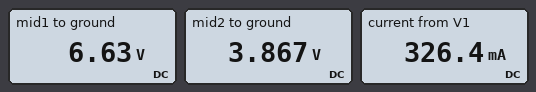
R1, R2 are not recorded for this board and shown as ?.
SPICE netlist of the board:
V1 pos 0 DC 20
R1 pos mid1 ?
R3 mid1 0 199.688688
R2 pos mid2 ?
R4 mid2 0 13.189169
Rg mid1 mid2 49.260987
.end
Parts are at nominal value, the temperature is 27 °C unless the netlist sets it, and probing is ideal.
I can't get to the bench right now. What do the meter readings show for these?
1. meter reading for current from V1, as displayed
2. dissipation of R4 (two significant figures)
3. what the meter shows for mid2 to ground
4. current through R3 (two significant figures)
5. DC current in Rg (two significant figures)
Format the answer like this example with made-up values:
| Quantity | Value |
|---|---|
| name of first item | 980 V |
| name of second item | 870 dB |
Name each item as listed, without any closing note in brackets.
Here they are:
| Quantity | Value |
|---|---|
| meter reading for current from V1, as displayed | 326.4 mA |
| dissipation of R4 | 1.1 W |
| what the meter shows for mid2 to ground | 3.867 V |
| current through R3 | 33 mA |
| DC current in Rg | 56 mA |
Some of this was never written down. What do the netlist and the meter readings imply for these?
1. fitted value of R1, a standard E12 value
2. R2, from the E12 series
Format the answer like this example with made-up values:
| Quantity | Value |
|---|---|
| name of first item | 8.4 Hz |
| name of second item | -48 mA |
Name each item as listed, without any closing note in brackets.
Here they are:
| Quantity | Value |
|---|---|
| fitted value of R1, a standard E12 value | 150 Ω |
| R2, from the E12 series | 68 Ω |
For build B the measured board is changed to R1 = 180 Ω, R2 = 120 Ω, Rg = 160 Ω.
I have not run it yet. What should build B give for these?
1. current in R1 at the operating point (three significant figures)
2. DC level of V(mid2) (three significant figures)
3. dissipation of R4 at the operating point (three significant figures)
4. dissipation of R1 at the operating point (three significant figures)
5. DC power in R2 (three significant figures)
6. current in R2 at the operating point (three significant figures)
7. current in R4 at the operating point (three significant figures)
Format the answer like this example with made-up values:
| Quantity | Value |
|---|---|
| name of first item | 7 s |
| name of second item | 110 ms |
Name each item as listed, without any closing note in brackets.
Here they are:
| Quantity | Value |
|---|---|
| current in R1 at the operating point | 69.5 mA |
| DC level of V(mid2) | 2.36 V |
| dissipation of R4 at the operating point | 423 mW |
| dissipation of R1 at the operating point | 870 mW |
| DC power in R2 | 2.59 W |
| current in R2 at the operating point | 147 mA |
| current in R4 at the operating point | 179 mA |
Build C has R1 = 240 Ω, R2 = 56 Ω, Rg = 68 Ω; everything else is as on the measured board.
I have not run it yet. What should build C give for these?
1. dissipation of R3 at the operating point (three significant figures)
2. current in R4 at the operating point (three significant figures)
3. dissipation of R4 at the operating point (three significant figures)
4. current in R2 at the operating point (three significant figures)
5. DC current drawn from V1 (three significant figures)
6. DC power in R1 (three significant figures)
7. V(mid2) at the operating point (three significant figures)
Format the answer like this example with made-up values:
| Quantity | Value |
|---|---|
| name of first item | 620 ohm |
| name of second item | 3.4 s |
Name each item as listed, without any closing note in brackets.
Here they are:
| Quantity | Value |
|---|---|
| dissipation of R3 at the operating point | 182 mW |
| current in R4 at the operating point | 312 mA |
| dissipation of R4 at the operating point | 1.28 W |
| current in R2 at the operating point | 284 mA |
| DC current drawn from V1 | 342 mA |
| DC power in R1 | 814 mW |
| V(mid2) at the operating point | 4.11 V |
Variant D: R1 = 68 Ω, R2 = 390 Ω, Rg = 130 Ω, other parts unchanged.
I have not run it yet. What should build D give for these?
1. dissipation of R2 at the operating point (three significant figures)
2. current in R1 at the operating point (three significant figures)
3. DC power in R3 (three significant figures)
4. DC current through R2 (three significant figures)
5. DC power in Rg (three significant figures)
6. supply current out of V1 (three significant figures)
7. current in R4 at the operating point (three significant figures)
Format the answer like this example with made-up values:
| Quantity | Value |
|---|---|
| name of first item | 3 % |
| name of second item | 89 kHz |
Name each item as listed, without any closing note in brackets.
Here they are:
| Quantity | Value |
|---|---|
| dissipation of R2 at the operating point | 869 mW |
| current in R1 at the operating point | 130 mA |
| DC power in R3 | 626 mW |
| DC current through R2 | 47.2 mA |
| DC power in Rg | 707 mW |
| supply current out of V1 | 177 mA |
| current in R4 at the operating point | 121 mA |
